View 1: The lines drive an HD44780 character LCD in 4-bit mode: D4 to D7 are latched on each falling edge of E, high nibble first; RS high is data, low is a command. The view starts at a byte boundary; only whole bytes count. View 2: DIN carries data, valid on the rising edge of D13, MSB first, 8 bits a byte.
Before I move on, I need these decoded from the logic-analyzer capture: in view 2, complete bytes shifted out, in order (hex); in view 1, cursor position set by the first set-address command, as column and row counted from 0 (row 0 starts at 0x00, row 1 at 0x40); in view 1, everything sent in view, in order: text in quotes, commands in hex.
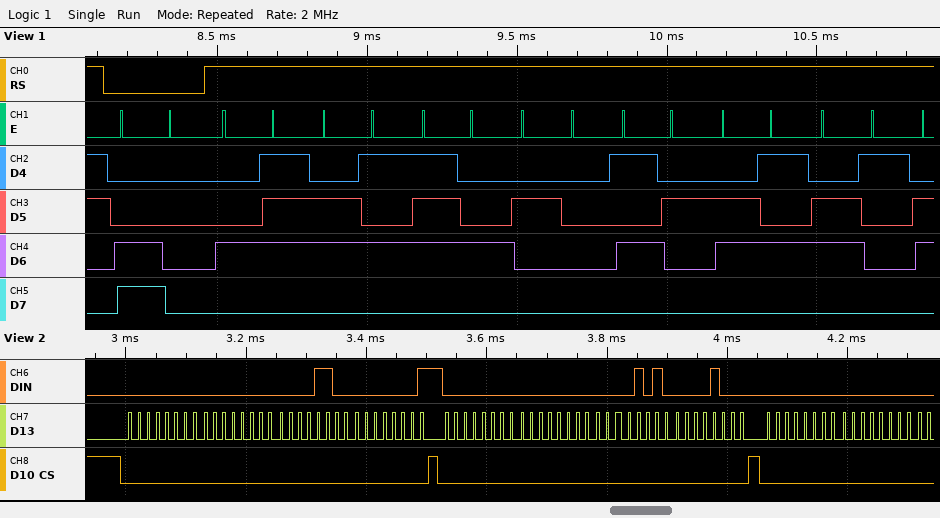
00 00 0C 01 00 00 0A 08 00 00
column 0, row 1
0xC0 "Get Rea"
